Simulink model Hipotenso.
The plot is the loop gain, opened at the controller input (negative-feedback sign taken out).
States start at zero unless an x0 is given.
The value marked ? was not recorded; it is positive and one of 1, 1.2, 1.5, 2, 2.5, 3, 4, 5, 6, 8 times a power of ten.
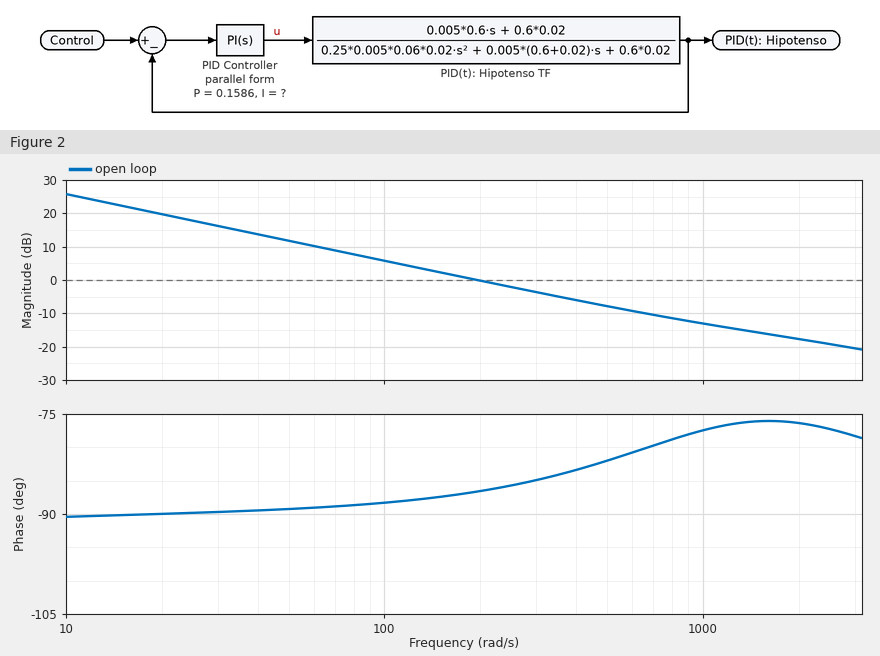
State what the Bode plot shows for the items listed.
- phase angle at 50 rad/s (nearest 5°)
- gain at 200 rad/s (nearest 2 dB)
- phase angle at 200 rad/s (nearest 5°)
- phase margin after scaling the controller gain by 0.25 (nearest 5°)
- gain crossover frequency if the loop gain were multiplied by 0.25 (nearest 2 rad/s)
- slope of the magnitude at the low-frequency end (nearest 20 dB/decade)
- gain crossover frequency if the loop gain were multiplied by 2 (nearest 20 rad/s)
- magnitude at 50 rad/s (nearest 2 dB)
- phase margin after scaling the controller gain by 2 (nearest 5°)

-90°
0 dB
-85°
90°
48 rad/s
-20 dB/decade
400 rad/s
12 dB
95°
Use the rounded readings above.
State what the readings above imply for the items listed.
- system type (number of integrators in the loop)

1
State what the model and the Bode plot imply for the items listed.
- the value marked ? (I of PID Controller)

200
